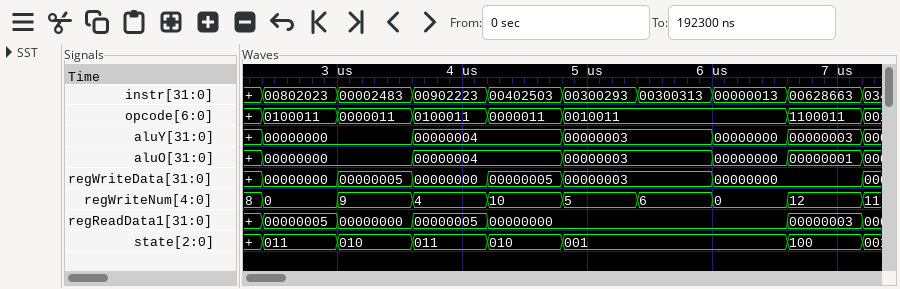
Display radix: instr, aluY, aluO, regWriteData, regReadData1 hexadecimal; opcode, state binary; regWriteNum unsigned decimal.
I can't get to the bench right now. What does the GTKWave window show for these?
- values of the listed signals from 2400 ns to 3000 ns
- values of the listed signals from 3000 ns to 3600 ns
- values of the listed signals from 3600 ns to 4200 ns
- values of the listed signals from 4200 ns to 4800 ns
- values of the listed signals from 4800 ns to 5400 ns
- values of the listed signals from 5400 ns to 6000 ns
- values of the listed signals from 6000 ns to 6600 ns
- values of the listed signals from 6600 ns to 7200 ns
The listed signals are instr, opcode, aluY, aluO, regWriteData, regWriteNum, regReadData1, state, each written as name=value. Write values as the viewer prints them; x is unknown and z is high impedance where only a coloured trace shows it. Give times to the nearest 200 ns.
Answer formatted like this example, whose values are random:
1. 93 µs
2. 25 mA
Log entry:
1. instr=00802023, opcode=0100011, aluY=00000000, aluO=00000000, regWriteData=00000000, regWriteNum=0, regReadData1=00000005, state=011
2. instr=00002483, opcode=0000011, aluY=00000000, aluO=00000000, regWriteData=00000005, regWriteNum=9, regReadData1=00000000, state=010
3. instr=00902223, opcode=0100011, aluY=00000004, aluO=00000004, regWriteData=00000000, regWriteNum=4, regReadData1=00000005, state=011
4. instr=00402503, opcode=0000011, aluY=00000004, aluO=00000004, regWriteData=00000005, regWriteNum=10, regReadData1=00000000, state=010
5. instr=00300293, opcode=0010011, aluY=00000003, aluO=00000003, regWriteData=00000003, regWriteNum=5, regReadData1=00000000, state=001
6. instr=00300313, opcode=0010011, aluY=00000003, aluO=00000003, regWriteData=00000003, regWriteNum=6, regReadData1=00000000, state=001
7. instr=00000013, opcode=0010011, aluY=00000000, aluO=00000000, regWriteData=00000000, regWriteNum=0, regReadData1=00000000, state=001
8. instr=00628663, opcode=1100011, aluY=00000003, aluO=00000001, regWriteData=00000000, regWriteNum=12, regReadData1=00000003, state=100
